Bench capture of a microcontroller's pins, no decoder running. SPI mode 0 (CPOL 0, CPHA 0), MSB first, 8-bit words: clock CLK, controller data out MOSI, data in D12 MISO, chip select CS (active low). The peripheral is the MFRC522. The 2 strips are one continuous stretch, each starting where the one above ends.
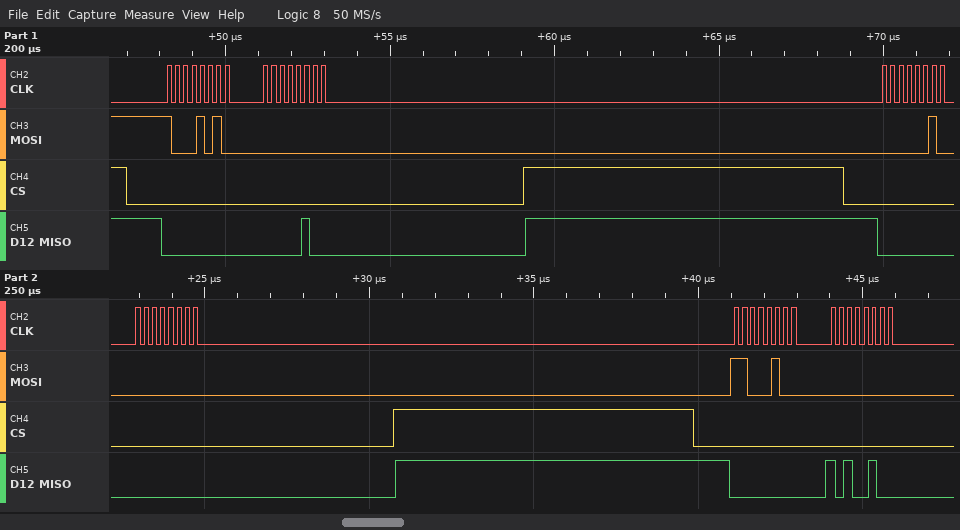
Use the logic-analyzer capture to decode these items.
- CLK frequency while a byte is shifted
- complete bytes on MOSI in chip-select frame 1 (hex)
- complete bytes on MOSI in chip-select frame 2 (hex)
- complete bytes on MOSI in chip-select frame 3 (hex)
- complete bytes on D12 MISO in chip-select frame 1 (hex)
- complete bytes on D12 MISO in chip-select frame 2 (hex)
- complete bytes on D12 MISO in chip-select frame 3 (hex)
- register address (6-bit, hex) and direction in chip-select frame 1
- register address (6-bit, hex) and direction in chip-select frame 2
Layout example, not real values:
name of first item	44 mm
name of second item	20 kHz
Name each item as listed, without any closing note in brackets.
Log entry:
CLK frequency while a byte is shifted	4 MHz
complete bytes on MOSI in chip-select frame 1	8A 00
complete bytes on MOSI in chip-select frame 2	02 00
complete bytes on MOSI in chip-select frame 3	C4 00
complete bytes on D12 MISO in chip-select frame 1	00 04
complete bytes on D12 MISO in chip-select frame 2	00 00
complete bytes on D12 MISO in chip-select frame 3	00 A4
register address (6-bit, hex) and direction in chip-select frame 1	0x05 read
register address (6-bit, hex) and direction in chip-select frame 2	0x01 write
